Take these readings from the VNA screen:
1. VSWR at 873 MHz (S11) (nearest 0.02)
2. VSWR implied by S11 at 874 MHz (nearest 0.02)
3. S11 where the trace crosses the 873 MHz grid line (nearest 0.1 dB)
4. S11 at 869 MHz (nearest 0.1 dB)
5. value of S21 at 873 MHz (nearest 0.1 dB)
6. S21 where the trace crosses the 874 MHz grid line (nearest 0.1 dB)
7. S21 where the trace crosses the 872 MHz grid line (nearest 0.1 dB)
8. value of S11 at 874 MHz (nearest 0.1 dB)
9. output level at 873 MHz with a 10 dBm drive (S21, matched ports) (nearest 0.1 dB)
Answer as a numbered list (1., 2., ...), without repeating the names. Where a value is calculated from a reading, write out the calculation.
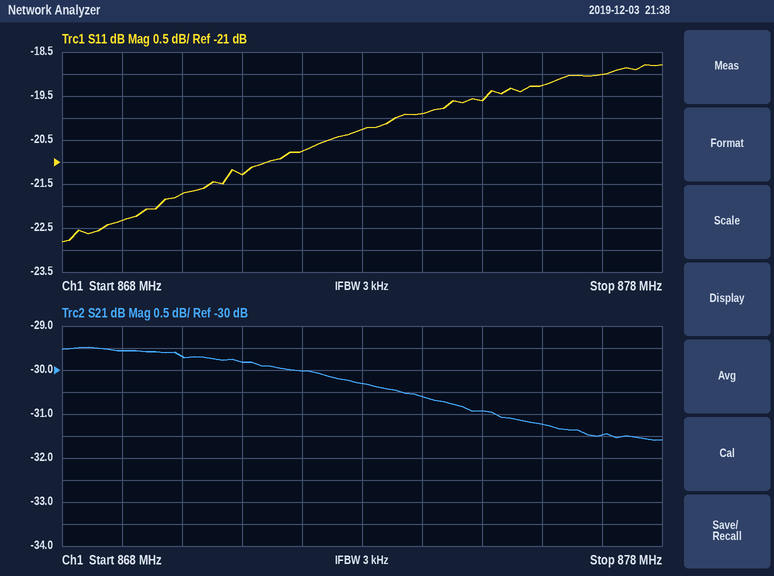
1. |Γ| = 10^(-20.3/20) = 0.0966; VSWR = (1 + 0.0966)/(1 − 0.0966) ≈ 1.21, so 1.22 to the nearest 0.02
2. |Γ| = 10^(-19.9/20) = 0.1012; VSWR = (1 + 0.1012)/(1 − 0.1012) ≈ 1.23, so 1.22 to the nearest 0.02
3. -20.3 dB
4. -22.3 dB
5. -30.3 dB
6. -30.6 dB
7. -30.0 dB
8. -19.9 dB
9. 10 dBm + (-30.3 dB) = -20.3 dBm
